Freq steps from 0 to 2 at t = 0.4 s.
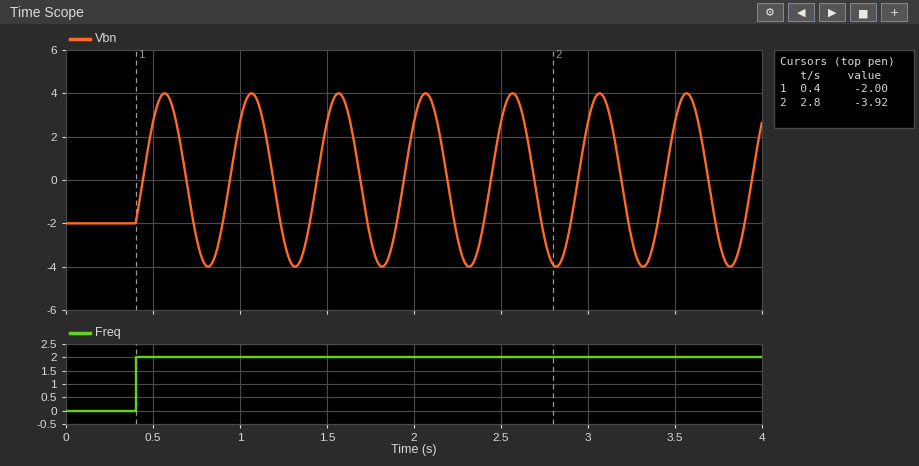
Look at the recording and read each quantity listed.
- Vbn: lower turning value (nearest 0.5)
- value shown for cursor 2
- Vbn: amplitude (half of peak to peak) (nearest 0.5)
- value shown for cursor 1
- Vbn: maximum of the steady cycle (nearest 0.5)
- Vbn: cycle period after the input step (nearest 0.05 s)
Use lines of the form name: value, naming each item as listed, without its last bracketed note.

Vbn: lower turning value: -4.0
value shown for cursor 2: -3.92
Vbn: amplitude (half of peak to peak): 4.0
value shown for cursor 1: -2.00
Vbn: maximum of the steady cycle: 4.0
Vbn: cycle period after the input step: 0.50 s
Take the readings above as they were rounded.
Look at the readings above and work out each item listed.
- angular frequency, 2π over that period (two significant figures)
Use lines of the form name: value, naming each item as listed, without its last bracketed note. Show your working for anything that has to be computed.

angular frequency, 2π over that period: 2π / 0.5 = 13 rad/s
